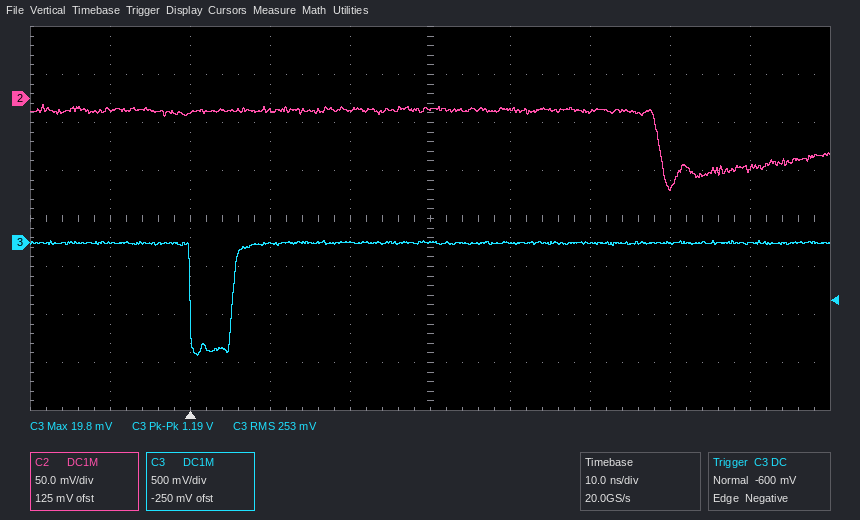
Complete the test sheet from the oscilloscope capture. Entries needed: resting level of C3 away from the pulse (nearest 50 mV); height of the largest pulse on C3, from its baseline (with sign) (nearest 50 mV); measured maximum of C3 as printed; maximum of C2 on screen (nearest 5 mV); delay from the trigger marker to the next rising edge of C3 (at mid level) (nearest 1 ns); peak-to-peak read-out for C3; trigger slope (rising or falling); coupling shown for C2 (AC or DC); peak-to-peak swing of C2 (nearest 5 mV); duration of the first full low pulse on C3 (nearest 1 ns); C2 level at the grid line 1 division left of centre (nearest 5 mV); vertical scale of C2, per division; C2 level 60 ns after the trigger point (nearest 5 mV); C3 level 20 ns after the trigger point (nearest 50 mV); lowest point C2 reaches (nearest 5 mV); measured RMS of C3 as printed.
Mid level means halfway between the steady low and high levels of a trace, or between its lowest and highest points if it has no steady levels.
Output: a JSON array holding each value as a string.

["0 mV", "-1.15 V", "19.8 mV", "-5 mV", "5 ns", "1.19 V", "falling", "DC", "90 mV", "5 ns", "-10 mV", "50 mV", "-90 mV", "0 mV", "-95 mV", "253 mV"]
